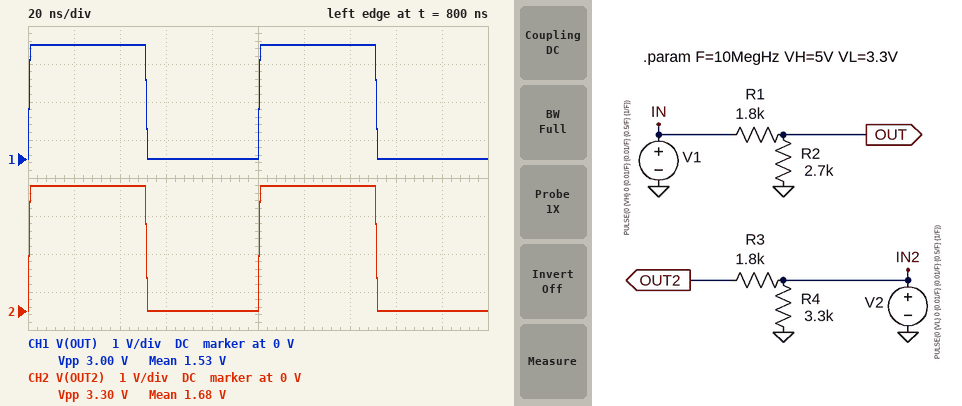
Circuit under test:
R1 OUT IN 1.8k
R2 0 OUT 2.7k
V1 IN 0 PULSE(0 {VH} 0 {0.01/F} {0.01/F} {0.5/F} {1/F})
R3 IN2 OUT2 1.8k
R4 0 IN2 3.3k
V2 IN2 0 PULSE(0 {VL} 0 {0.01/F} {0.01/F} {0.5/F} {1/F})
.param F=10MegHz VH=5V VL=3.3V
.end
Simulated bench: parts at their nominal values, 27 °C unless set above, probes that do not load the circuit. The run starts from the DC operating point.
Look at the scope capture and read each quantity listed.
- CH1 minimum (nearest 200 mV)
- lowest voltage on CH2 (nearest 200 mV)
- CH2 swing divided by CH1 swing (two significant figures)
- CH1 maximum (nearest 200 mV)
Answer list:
0 V
0 V
1.1
3.0 V
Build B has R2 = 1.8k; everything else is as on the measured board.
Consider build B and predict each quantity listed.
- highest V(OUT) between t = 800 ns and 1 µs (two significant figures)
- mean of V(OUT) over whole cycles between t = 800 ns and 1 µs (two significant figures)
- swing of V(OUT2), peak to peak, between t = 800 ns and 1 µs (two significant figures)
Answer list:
2.5 V
1.3 V
3.3 V
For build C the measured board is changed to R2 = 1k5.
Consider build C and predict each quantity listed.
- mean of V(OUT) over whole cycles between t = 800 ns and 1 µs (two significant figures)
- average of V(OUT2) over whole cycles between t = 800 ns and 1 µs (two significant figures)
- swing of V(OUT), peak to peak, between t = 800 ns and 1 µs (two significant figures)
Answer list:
1.2 V
1.7 V
2.3 V
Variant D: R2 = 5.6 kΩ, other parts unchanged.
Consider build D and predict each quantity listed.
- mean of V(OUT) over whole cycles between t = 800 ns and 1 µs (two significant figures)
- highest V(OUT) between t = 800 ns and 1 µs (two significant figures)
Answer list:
1.9 V
3.8 V
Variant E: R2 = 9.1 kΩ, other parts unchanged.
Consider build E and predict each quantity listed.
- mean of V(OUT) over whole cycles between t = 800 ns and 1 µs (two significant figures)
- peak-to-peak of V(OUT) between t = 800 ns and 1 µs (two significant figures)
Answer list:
2.1 V
4.2 V
